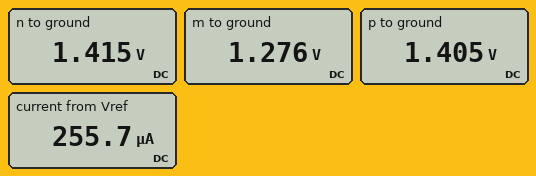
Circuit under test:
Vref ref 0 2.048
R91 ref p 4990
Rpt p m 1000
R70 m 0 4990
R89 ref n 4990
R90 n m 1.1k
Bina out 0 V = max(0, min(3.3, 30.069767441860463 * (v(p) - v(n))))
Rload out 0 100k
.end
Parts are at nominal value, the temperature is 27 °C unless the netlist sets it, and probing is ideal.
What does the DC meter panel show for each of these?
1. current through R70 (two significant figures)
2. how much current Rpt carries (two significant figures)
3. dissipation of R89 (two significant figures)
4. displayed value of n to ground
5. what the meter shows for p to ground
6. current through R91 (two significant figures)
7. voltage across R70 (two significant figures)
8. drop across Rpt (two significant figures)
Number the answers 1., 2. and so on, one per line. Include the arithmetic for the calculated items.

1. (1.276 V) / 4.99 kΩ = 260 µA
2. (1.405 V - 1.276 V) / 1 kΩ = 130 µA
3. (2.048 V - 1.415 V)^2 / 4.99 kΩ = 80 µW
4. 1.415 V
5. 1.405 V
6. (2.048 V - 1.405 V) / 4.99 kΩ = 130 µA
7. 1.276 V = 1.3 V
8. 1.405 V - 1.276 V = 130 mV
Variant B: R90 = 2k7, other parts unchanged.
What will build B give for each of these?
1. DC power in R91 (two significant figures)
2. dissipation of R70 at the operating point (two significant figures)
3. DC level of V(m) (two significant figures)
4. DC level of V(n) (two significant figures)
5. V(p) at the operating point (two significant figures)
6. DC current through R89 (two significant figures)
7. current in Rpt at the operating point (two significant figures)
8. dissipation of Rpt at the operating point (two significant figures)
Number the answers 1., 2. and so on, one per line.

1. 95 µW
2. 300 µW
3. 1.2 V
4. 1.5 V
5. 1.4 V
6. 110 µA
7. 140 µA
8. 19 µW
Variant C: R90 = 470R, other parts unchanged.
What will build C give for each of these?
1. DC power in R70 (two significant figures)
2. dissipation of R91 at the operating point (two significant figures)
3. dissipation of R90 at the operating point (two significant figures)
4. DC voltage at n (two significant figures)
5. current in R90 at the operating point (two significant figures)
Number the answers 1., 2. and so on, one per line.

1. 340 µW
2. 77 µW
3. 8.8 µW
4. 1.4 V
5. 140 µA
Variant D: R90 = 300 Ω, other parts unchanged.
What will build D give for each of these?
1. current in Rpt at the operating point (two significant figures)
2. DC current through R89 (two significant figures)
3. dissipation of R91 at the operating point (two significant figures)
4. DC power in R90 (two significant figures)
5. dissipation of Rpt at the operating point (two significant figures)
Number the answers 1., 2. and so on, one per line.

1. 120 µA
2. 140 µA
3. 76 µW
4. 5.8 µW
5. 15 µW
